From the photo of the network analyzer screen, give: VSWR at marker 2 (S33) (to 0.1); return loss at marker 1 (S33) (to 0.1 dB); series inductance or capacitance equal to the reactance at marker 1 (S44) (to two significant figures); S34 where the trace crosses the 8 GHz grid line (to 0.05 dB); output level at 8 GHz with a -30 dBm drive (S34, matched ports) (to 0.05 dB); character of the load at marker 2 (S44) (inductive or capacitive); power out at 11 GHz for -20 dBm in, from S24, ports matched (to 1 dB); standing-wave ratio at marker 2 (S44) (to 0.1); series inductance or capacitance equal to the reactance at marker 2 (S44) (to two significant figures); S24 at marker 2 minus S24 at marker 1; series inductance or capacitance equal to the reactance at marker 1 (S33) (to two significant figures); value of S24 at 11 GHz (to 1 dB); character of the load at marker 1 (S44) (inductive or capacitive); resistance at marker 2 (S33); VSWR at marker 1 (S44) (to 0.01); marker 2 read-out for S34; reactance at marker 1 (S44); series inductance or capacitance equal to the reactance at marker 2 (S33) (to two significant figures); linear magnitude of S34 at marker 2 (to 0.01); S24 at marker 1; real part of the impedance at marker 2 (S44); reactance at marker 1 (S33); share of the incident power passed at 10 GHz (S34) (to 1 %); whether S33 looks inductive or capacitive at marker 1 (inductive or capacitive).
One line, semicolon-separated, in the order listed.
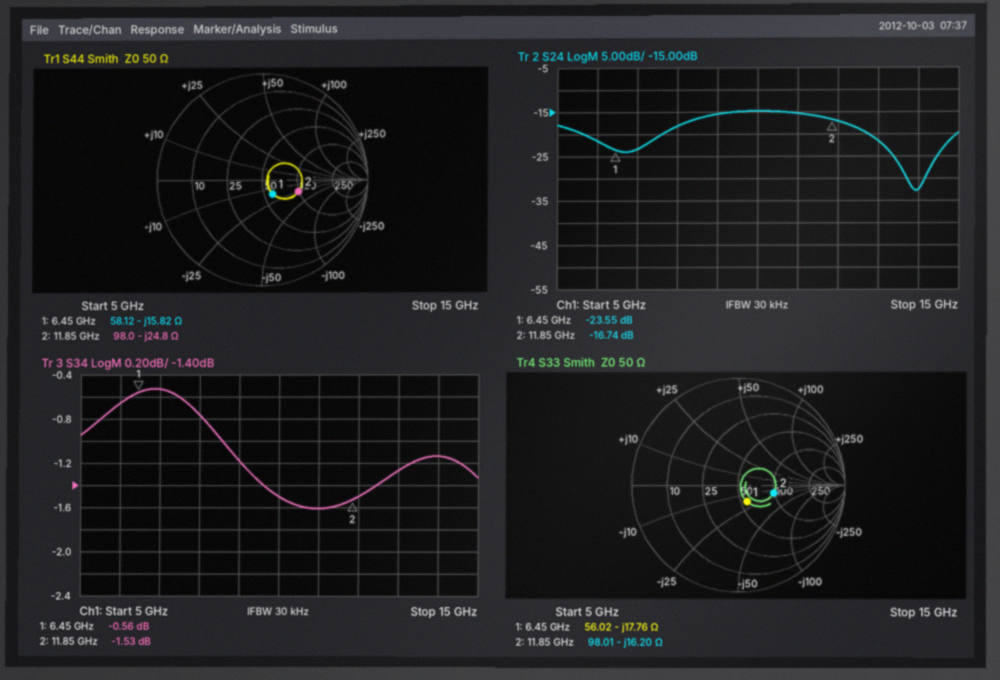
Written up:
2.0; 15.2 dB; 1.6 pF; -0.75 dB; -30.75 dBm; capacitive; -35 dBm; 2.1; 540 fF; 6.81 dB; 1.4 pF; -15 dB; capacitive; 98.01 Ω; 1.39; -1.53 dB; -15.82 Ω; 830 fF; 0.84; -23.55 dB; 98.0 Ω; -17.76 Ω; 71 %; capacitive
